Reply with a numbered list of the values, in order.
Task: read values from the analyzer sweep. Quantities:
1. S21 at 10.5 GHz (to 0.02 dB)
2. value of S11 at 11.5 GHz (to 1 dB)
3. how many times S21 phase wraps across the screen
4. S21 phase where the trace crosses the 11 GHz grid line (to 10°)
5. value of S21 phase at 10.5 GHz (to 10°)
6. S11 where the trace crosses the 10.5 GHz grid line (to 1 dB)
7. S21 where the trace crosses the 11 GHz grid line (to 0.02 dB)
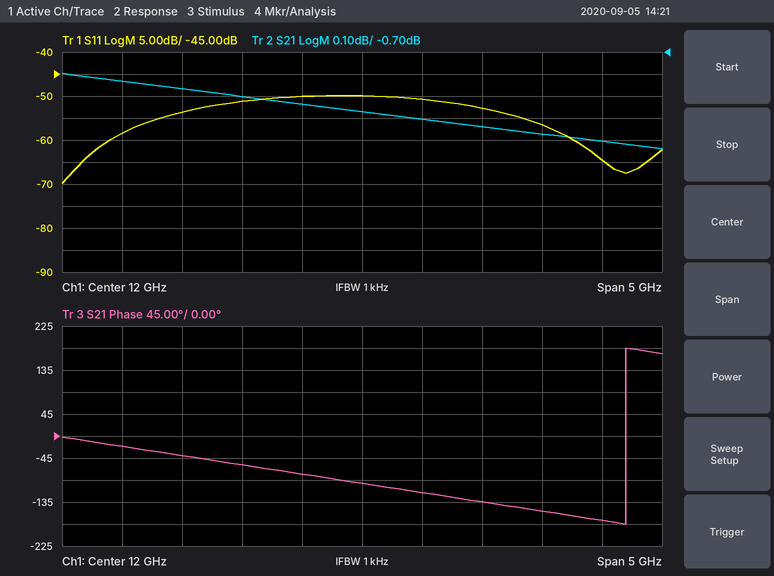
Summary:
1. -0.86 dB
2. -50 dB
3. 1
4. -60°
5. -40°
6. -54 dB
7. -0.90 dB
